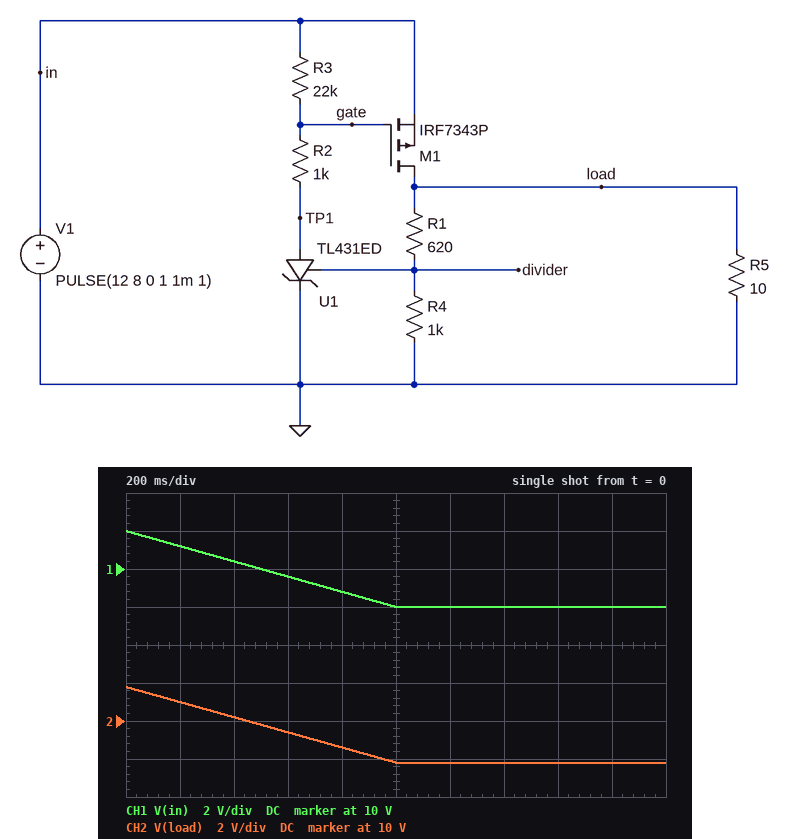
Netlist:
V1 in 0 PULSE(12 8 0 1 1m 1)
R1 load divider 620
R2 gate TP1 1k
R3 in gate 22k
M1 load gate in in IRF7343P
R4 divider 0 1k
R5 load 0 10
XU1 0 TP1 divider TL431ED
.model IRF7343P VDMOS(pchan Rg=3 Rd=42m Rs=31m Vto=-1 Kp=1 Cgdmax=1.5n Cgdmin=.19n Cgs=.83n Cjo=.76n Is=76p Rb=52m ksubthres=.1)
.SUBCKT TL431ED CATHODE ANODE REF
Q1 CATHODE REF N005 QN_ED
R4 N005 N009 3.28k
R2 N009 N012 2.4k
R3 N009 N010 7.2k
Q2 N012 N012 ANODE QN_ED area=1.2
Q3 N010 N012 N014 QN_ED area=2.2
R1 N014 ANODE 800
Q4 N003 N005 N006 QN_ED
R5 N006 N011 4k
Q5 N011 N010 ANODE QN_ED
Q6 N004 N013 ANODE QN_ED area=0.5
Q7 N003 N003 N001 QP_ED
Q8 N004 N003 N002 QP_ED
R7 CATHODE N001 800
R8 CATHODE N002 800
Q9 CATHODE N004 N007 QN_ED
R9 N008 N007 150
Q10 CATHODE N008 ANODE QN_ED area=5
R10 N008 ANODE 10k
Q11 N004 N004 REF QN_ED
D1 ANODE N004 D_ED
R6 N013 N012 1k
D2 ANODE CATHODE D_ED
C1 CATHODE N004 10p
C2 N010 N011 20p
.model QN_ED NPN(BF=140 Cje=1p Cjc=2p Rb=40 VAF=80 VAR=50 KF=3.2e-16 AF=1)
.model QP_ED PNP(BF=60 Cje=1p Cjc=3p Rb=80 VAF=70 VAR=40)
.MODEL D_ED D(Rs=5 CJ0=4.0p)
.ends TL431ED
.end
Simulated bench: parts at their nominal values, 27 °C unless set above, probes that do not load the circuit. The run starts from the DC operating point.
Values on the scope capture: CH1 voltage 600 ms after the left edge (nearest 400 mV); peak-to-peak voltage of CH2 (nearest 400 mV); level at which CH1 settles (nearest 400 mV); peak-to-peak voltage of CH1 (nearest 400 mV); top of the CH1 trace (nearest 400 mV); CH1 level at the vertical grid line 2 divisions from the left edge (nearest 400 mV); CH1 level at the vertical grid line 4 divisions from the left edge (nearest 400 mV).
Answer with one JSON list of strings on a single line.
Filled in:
["9.6 V", "4.0 V", "8.0 V", "4.0 V", "12.0 V", "10.4 V", "8.8 V"]
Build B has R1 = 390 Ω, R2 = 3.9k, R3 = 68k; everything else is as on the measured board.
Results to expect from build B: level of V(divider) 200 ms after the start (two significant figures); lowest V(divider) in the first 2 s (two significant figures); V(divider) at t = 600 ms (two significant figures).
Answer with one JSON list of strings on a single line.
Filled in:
["1.7 V", "1.4 V", "1.6 V"]
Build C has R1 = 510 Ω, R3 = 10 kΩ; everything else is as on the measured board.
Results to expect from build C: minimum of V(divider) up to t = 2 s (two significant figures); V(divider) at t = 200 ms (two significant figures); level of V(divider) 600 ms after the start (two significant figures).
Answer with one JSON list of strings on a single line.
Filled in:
["1.3 V", "1.5 V", "1.4 V"]
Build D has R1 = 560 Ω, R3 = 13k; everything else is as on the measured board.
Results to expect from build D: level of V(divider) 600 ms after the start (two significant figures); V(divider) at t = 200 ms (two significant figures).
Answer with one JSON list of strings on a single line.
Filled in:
["1.4 V", "1.5 V"]
